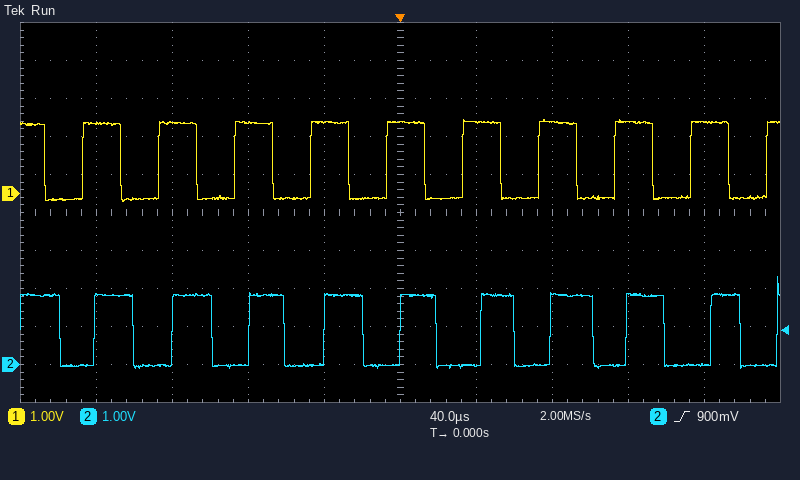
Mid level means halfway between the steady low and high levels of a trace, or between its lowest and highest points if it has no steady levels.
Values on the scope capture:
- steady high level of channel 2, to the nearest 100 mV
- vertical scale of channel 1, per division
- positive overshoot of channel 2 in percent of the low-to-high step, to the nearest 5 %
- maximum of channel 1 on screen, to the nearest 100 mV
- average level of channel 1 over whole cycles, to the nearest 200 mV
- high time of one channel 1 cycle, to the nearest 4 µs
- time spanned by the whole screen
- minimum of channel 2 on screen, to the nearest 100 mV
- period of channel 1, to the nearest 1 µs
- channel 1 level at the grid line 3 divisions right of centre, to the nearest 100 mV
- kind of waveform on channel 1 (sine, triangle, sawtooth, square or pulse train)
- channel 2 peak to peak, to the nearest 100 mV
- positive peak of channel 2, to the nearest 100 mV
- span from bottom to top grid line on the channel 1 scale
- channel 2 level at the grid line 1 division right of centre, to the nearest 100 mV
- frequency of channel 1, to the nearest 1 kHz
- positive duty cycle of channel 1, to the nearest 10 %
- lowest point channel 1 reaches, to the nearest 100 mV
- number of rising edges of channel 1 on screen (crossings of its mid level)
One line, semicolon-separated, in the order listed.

1.8 V; 1 V; 25 %; 1.9 V; 800 mV; 20 µs; 400 µs; -100 mV; 40 µs; 1.9 V; square; 2.4 V; 2.3 V; 10 V; 0.0 V; 25 kHz; 50 %; -200 mV; 10
